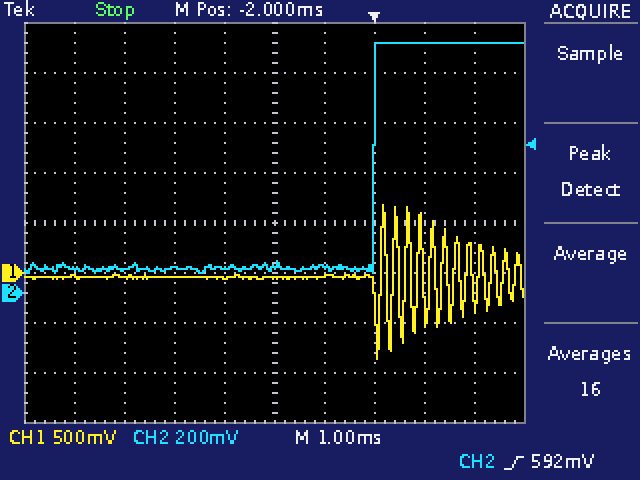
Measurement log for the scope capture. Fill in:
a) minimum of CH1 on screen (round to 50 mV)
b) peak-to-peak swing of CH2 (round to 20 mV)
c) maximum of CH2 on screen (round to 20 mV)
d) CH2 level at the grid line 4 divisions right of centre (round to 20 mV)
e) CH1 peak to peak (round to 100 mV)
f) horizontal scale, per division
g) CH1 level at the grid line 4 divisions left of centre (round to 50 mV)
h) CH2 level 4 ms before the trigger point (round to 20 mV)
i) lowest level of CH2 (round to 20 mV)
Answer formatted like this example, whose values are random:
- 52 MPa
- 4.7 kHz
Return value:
- -850 mV
- 920 mV
- 1.00 V
- 1.00 V
- 1.50 V
- 1 ms
- -50 mV
- 100 mV
- 80 mV
